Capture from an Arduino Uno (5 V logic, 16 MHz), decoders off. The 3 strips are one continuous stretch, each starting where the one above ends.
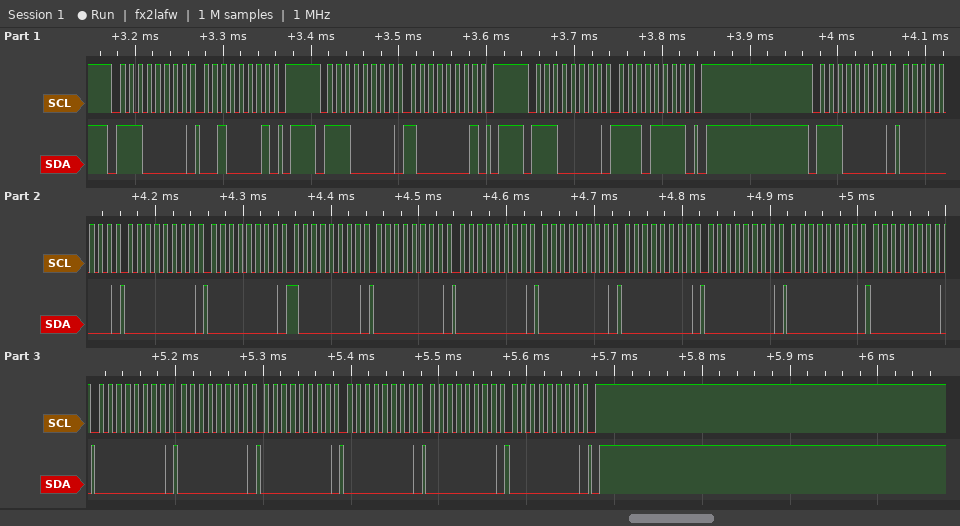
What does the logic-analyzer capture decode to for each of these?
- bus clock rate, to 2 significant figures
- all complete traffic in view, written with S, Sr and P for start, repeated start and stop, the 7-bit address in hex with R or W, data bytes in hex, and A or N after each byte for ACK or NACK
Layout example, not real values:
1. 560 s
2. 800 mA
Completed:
1. 100 kHz
2. S 70W A 21 A P S 70W A 81 A P S 70W A EF A P S 70W A 00 A 00 A 00 A 80 A 00 A 00 A 00 A 00 A 00 A 00 A 00 A 00 A 00 A 00 A 00 A 00 A 00 A P
